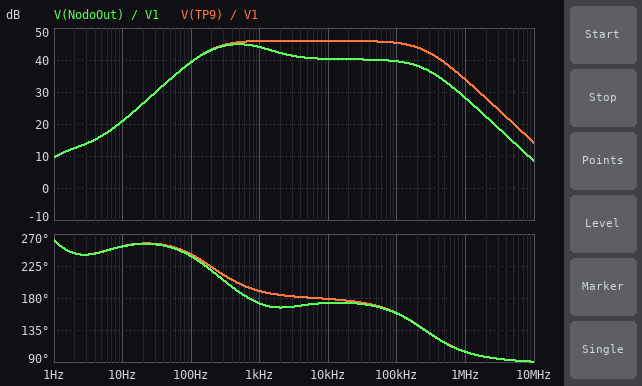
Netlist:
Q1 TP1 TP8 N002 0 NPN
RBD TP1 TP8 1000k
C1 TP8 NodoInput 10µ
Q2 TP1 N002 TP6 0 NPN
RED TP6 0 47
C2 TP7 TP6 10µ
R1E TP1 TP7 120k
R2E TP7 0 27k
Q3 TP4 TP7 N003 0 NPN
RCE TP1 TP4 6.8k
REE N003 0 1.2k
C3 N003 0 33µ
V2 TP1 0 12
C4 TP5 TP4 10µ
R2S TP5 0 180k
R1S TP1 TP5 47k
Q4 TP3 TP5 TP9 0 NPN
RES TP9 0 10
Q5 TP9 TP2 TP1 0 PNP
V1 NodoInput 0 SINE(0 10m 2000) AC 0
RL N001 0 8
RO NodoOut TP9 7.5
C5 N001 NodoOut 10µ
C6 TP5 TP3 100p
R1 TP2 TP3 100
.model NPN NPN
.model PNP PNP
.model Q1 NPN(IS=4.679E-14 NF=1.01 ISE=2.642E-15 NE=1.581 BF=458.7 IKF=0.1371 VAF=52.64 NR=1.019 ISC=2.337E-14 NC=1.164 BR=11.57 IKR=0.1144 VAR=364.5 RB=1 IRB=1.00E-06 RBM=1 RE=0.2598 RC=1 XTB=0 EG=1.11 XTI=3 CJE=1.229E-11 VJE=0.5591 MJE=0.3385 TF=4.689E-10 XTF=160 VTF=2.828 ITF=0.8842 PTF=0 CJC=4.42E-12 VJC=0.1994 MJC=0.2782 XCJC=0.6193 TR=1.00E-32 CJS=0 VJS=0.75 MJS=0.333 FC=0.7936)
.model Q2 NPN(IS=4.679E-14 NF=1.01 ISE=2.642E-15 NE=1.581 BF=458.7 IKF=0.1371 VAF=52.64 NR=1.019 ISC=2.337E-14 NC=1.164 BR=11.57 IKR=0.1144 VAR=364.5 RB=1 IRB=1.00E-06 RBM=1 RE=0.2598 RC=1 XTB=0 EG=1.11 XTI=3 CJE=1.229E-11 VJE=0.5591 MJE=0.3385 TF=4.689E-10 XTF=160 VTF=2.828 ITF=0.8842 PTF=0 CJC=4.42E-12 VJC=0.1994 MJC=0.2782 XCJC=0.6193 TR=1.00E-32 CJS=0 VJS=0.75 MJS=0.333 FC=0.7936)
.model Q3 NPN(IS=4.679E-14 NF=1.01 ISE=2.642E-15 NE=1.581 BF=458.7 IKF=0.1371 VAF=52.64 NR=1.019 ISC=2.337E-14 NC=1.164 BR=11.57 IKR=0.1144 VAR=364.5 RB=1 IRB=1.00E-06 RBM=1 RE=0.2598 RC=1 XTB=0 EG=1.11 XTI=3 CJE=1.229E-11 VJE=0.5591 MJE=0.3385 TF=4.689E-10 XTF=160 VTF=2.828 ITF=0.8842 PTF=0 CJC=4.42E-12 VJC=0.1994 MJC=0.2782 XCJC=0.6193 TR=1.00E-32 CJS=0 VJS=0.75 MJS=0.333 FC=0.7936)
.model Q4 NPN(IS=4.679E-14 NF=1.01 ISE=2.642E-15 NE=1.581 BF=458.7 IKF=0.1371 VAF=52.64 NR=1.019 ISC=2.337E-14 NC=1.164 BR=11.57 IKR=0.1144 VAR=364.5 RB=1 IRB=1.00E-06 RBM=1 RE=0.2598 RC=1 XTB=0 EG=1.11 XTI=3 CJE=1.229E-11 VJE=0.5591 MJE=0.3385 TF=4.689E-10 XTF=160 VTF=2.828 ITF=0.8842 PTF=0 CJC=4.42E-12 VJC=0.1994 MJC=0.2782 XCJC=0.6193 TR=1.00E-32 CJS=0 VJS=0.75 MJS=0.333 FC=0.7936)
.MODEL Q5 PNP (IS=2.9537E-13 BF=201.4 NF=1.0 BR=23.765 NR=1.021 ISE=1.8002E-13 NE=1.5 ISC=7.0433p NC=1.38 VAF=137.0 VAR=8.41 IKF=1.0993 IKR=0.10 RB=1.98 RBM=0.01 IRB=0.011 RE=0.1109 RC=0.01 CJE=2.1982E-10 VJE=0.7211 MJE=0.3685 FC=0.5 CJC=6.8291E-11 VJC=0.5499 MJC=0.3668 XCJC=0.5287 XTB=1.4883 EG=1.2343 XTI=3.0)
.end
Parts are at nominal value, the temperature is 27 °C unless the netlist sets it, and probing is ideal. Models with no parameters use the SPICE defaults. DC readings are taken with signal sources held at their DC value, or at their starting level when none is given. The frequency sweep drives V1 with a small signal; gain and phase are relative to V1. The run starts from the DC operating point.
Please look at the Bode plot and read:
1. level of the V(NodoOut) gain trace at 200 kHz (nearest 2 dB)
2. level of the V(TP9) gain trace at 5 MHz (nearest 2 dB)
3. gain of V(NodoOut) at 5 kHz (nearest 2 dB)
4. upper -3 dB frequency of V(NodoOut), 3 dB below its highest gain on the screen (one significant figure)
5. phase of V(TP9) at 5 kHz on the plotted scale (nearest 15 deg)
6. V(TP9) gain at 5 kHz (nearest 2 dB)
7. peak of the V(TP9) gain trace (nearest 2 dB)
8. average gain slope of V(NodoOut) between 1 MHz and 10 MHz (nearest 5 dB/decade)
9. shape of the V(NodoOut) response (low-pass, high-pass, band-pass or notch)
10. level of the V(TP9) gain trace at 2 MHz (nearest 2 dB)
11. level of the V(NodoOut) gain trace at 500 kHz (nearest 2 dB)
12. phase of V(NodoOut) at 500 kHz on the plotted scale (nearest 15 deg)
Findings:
38 dB
20 dB
40 dB
2 kHz
180 deg
46 dB
46 dB
-20 dB/decade
band-pass
28 dB
34 dB
120 deg
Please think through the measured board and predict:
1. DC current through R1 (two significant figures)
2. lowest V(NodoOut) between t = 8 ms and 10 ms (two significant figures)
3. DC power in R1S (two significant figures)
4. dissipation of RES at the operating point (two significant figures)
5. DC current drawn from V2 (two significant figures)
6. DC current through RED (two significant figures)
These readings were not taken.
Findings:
6.3 mA
5.0 V
500 µW
4.0 W
710 mA
71 mA
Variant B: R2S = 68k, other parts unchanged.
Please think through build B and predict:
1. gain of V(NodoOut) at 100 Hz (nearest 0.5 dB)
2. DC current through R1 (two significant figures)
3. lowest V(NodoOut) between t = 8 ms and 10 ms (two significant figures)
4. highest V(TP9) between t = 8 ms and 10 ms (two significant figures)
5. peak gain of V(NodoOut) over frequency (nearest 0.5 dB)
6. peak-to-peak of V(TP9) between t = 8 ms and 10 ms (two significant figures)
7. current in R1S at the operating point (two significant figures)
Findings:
39.0 dB
4.9 mA
3.6 V
6.6 V
44.5 dB
3.7 V
130 µA
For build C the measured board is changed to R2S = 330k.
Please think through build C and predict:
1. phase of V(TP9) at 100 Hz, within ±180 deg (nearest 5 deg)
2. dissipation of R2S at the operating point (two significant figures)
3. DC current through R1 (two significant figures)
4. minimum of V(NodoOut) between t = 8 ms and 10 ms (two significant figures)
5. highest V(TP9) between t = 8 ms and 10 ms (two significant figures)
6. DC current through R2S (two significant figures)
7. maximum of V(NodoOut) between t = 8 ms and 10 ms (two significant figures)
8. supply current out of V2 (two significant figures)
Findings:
-120 deg
180 µW
6.8 mA
5.5 V
8.7 V
23 µA
8.1 V
760 mA
